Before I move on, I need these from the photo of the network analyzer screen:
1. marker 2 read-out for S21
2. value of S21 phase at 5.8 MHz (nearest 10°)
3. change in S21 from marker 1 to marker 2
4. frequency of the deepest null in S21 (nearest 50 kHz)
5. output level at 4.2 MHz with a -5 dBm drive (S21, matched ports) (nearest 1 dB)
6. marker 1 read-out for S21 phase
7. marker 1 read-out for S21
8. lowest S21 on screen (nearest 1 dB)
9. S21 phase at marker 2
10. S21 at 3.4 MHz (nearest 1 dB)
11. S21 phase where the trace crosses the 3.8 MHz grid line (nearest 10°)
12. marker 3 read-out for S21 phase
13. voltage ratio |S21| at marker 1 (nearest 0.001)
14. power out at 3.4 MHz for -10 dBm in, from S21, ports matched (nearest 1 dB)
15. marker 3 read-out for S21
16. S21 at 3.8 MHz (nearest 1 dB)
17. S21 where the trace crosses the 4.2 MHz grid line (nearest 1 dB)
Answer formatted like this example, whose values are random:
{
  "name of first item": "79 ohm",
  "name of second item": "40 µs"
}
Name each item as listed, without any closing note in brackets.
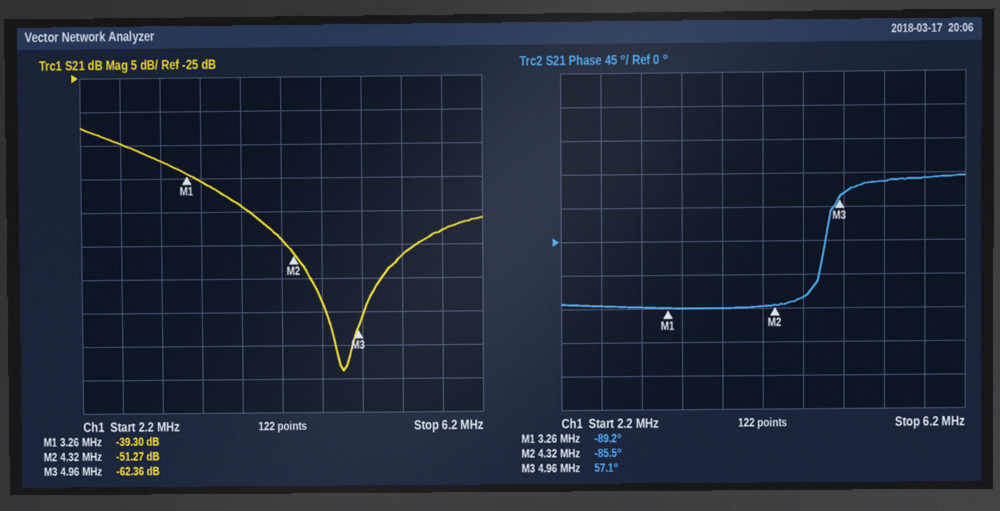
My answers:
{
  "marker 2 read-out for S21": "-51.27 dB",
  "value of S21 phase at 5.8 MHz": "80°",
  "change in S21 from marker 1 to marker 2": "-11.97 dB",
  "frequency of the deepest null in S21": "4.80 MHz",
  "output level at 4.2 MHz with a -5 dBm drive (S21, matched ports)": "-54 dBm",
  "marker 1 read-out for S21 phase": "-89.2°",
  "marker 1 read-out for S21": "-39.30 dB",
  "lowest S21 on screen": "-69 dB",
  "S21 phase at marker 2": "-85.5°",
  "S21 at 3.4 MHz": "-40 dB",
  "S21 phase where the trace crosses the 3.8 MHz grid line": "-90°",
  "marker 3 read-out for S21 phase": "57.1°",
  "voltage ratio |S21| at marker 1": "0.011",
  "power out at 3.4 MHz for -10 dBm in, from S21, ports matched": "-50 dBm",
  "marker 3 read-out for S21": "-62.36 dB",
  "S21 at 3.8 MHz": "-44 dB",
  "S21 where the trace crosses the 4.2 MHz grid line": "-49 dB"
}
